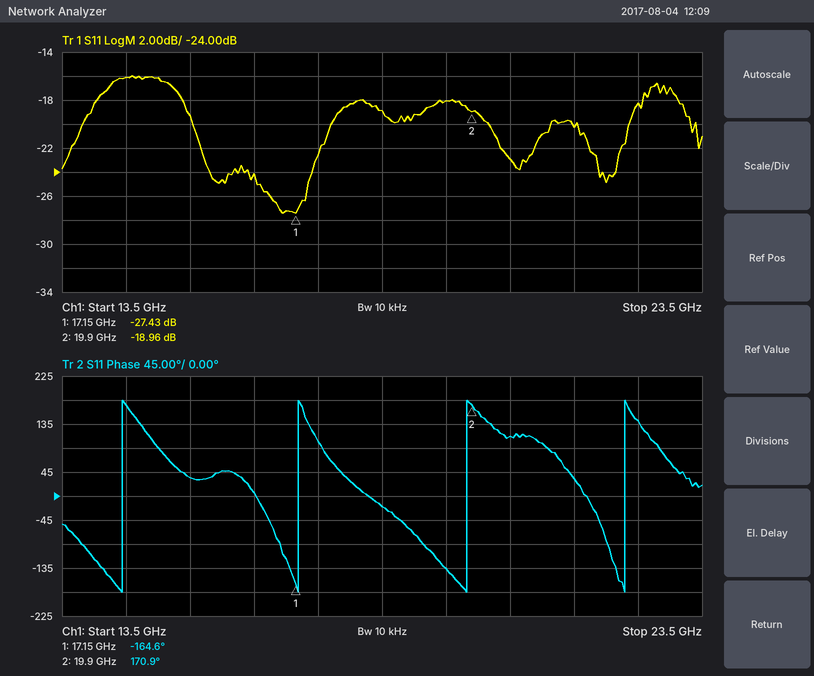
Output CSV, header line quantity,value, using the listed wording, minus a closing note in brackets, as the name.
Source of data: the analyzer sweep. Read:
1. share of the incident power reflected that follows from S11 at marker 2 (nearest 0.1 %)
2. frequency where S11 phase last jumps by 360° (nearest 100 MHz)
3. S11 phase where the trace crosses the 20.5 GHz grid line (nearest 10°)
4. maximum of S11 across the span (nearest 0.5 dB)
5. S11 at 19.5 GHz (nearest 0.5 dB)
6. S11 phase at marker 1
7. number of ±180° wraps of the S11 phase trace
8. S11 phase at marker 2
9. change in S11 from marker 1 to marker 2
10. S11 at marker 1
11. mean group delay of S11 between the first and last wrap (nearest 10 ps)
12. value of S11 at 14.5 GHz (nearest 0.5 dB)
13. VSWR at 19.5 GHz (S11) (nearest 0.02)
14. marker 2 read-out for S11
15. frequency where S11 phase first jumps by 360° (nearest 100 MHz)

quantity,value
share of the incident power reflected that follows from S11 at marker 2,1.3 %
frequency where S11 phase last jumps by 360°,22.3 GHz
S11 phase where the trace crosses the 20.5 GHz grid line,110°
maximum of S11 across the span,-16.0 dB
S11 at 19.5 GHz,-18.0 dB
S11 phase at marker 1,-164.6°
number of ±180° wraps of the S11 phase trace,4
S11 phase at marker 2,170.9°
change in S11 from marker 1 to marker 2,8.47 dB
S11 at marker 1,-27.43 dB
mean group delay of S11 between the first and last wrap,380 ps
value of S11 at 14.5 GHz,-16.0 dB
VSWR at 19.5 GHz (S11),1.28
marker 2 read-out for S11,-18.96 dB
frequency where S11 phase first jumps by 360°,14.4 GHz
